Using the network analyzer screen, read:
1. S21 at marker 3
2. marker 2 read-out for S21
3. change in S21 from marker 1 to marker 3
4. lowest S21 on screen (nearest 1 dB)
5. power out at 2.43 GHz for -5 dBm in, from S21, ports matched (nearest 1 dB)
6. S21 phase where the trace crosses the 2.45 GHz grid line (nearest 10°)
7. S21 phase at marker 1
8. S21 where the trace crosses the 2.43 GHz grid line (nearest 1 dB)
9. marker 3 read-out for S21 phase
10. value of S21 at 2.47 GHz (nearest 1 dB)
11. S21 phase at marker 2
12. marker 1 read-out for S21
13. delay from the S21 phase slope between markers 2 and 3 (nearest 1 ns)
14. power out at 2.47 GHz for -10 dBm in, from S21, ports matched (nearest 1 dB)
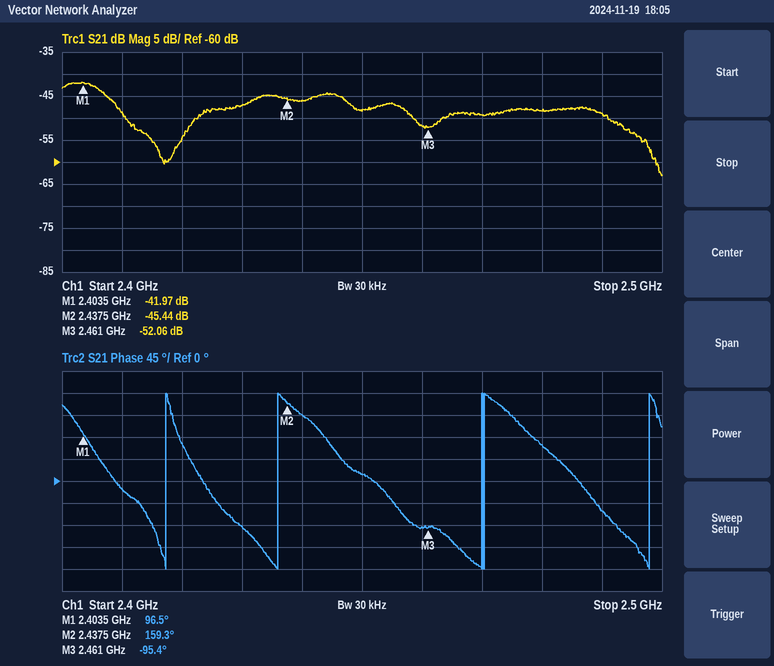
-52.06 dB
-45.44 dB
-10.09 dB
-63 dB
-52 dBm
10°
96.5°
-47 dB
-95.4°
-49 dB
159.3°
-41.97 dB
30 ns
-59 dBm
